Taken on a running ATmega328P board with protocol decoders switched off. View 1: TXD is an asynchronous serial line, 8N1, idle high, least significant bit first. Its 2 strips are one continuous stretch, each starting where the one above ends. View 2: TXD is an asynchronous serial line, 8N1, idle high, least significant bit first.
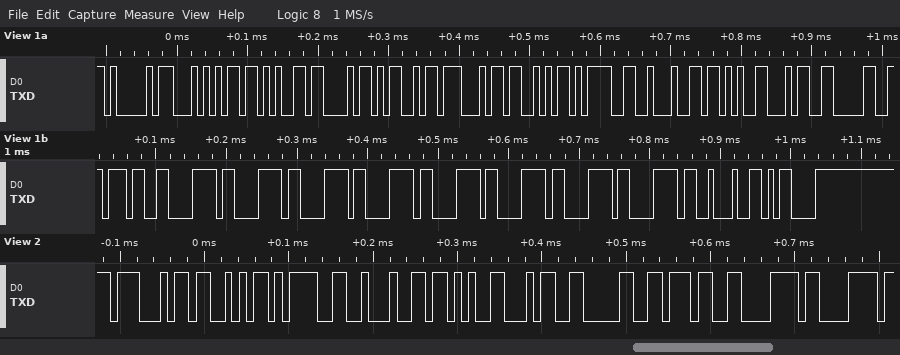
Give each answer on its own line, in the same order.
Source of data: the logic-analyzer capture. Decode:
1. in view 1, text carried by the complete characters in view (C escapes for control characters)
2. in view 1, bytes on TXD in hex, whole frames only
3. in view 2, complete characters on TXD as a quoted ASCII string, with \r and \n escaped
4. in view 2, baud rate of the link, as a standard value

"AT+CMGS=\"+407xxxxxxxx\"\r"
41 54 2B 43 4D 47 53 3D 22 2B 34 30 37 78 78 78 78 78 78 78 78 22 0D
"GS=\"+407xx"
115200 baud
